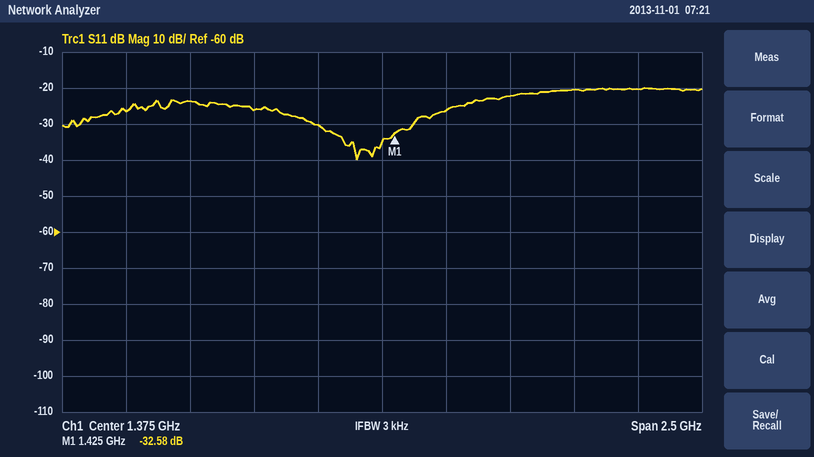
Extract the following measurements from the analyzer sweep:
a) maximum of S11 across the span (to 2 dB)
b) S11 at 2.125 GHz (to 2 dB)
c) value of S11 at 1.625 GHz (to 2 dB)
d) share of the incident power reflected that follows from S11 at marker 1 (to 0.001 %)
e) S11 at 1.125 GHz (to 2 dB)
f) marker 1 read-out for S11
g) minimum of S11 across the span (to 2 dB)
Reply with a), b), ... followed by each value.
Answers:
a) -20 dB
b) -20 dB
c) -26 dB
d) 0.055 %
e) -30 dB
f) -32.58 dB
g) -40 dB
